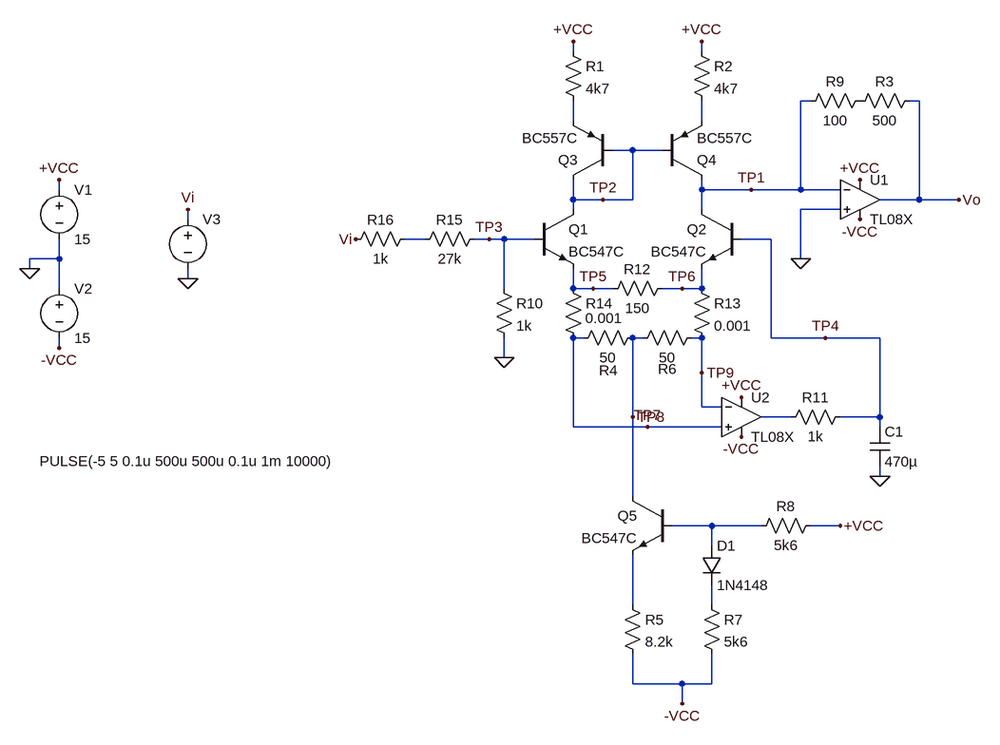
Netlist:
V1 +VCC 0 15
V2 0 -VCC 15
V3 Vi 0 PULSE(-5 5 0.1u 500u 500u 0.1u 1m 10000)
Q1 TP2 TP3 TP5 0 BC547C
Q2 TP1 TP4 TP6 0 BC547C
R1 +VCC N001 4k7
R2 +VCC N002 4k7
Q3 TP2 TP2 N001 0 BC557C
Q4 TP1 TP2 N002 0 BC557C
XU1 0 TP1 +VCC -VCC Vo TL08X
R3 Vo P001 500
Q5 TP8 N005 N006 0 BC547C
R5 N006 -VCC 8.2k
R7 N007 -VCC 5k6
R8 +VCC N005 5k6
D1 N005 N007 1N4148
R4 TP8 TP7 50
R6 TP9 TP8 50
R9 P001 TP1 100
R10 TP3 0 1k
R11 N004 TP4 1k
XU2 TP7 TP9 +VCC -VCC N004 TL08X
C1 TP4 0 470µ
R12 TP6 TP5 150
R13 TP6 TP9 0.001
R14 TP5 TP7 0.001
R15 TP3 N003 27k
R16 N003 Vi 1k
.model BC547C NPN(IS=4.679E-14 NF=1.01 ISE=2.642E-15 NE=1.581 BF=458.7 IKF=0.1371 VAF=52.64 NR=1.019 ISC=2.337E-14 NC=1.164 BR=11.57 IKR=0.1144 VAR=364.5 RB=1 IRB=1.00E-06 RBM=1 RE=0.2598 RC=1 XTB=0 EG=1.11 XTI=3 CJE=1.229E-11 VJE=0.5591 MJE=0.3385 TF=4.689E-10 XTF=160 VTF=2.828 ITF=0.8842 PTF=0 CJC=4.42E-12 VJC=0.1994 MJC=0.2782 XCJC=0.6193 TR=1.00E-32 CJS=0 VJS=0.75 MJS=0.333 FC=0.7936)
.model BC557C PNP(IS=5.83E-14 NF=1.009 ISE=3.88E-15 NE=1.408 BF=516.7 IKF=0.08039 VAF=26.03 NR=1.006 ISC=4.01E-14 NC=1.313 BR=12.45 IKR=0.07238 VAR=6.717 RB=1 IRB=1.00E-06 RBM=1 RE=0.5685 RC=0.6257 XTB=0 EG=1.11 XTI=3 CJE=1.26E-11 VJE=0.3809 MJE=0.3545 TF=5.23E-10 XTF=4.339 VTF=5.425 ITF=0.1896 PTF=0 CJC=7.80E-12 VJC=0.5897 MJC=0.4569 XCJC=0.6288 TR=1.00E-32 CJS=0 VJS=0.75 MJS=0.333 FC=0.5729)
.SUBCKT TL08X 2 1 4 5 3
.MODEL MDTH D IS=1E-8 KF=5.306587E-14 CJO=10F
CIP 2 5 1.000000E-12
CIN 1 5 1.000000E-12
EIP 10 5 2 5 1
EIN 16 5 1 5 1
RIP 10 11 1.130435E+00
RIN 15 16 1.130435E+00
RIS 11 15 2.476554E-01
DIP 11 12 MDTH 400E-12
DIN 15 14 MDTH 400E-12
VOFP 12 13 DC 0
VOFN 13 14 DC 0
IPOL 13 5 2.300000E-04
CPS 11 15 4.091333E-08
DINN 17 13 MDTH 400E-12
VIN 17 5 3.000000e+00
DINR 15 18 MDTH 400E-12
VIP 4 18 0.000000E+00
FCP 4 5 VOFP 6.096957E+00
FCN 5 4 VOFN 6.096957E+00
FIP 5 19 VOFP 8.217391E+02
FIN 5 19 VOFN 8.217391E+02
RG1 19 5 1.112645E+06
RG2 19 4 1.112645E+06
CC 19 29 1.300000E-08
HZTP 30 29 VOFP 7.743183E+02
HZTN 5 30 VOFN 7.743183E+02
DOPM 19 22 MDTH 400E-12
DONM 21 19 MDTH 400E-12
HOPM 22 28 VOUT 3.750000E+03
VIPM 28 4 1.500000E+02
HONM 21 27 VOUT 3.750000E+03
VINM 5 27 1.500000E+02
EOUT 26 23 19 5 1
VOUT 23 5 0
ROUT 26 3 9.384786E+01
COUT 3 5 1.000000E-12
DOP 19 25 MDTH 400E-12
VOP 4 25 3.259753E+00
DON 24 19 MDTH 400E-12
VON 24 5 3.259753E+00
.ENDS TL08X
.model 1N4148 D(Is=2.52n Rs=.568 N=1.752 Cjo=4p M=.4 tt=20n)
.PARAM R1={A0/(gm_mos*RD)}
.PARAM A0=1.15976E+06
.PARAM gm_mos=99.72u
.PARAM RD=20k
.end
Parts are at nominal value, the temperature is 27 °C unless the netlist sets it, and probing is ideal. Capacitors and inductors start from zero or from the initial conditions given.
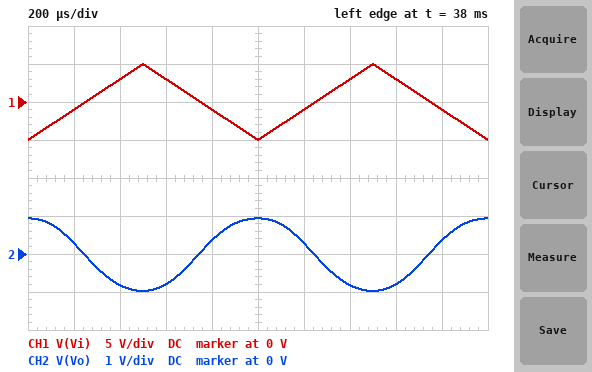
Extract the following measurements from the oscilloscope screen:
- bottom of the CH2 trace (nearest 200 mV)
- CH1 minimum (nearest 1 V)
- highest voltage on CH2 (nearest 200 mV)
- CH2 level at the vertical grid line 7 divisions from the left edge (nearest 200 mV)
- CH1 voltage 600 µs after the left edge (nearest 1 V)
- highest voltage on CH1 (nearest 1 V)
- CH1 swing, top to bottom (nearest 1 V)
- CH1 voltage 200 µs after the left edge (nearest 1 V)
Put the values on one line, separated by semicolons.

-1.0 V; -5 V; 1.0 V; -800 mV; 3 V; 5 V; 10 V; -1 V
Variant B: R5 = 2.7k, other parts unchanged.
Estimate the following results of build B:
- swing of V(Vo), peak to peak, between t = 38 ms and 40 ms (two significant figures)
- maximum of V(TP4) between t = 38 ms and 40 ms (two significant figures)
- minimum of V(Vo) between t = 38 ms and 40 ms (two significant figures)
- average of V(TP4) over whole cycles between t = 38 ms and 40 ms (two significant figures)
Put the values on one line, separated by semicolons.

3.1 V; 1.8 mV; -810 mV; -4.1 mV
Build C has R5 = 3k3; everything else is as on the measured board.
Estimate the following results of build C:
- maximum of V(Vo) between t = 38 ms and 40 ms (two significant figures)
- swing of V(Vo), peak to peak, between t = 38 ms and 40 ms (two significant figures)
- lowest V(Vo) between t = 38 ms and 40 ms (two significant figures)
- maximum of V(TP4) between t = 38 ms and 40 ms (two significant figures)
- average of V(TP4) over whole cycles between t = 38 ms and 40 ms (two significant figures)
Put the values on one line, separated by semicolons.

2.0 V; 3.4 V; -1.3 V; 4.0 mV; -1.9 mV
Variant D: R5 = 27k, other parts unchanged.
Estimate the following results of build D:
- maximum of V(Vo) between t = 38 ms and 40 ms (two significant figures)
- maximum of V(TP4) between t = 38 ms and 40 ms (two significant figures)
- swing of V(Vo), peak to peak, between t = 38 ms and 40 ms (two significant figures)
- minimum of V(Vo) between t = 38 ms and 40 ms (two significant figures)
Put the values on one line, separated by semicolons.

250 mV; 11 mV; 540 mV; -290 mV
